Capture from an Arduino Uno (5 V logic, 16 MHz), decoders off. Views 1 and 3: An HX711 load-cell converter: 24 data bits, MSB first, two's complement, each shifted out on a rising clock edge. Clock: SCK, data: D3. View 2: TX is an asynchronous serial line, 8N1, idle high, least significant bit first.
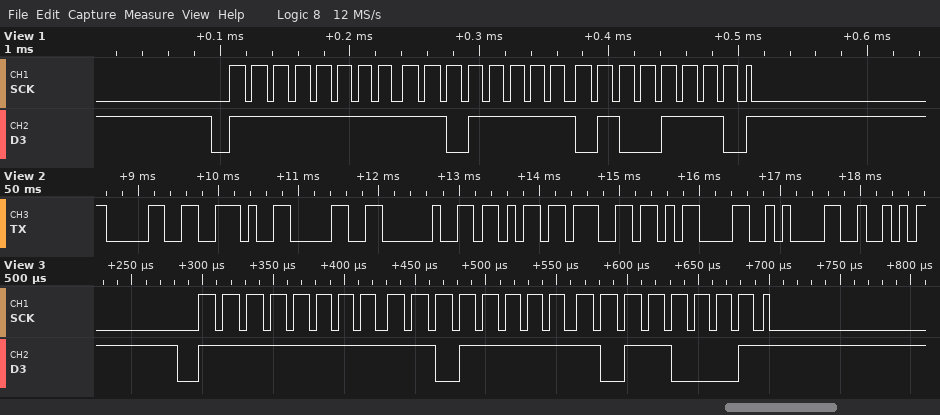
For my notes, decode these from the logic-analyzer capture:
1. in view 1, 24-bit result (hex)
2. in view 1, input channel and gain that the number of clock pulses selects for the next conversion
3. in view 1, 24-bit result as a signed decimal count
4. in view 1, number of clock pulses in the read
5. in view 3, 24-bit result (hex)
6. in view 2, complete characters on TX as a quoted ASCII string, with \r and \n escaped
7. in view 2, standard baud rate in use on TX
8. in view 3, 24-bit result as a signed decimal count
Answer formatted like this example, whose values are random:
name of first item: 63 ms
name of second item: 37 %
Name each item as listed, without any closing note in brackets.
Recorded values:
in view 1, 24-bit result: 0xFFDF4E
in view 1, input channel and gain that the number of clock pulses selects for the next conversion: channel A, gain 128
in view 1, 24-bit result as a signed decimal count: -8370
in view 1, number of clock pulses in the read: 25
in view 3, 24-bit result: 0xFFDFB1
in view 2, complete characters on TX as a quoted ASCII string, with \r and \n escaped: "0.0 kg\r\nR"
in view 2, standard baud rate in use on TX: 9600 baud
in view 3, 24-bit result as a signed decimal count: -8271
